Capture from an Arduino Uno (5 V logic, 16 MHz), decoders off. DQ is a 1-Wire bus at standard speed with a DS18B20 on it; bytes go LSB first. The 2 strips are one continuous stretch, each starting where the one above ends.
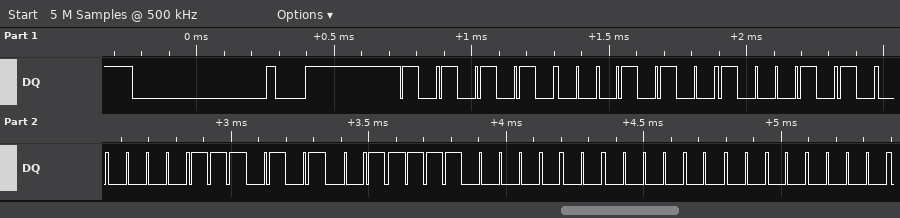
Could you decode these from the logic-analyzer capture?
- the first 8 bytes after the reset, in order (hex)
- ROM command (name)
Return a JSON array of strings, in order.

["55 28 51 E0 CA 07 00 00", "Match ROM"]
